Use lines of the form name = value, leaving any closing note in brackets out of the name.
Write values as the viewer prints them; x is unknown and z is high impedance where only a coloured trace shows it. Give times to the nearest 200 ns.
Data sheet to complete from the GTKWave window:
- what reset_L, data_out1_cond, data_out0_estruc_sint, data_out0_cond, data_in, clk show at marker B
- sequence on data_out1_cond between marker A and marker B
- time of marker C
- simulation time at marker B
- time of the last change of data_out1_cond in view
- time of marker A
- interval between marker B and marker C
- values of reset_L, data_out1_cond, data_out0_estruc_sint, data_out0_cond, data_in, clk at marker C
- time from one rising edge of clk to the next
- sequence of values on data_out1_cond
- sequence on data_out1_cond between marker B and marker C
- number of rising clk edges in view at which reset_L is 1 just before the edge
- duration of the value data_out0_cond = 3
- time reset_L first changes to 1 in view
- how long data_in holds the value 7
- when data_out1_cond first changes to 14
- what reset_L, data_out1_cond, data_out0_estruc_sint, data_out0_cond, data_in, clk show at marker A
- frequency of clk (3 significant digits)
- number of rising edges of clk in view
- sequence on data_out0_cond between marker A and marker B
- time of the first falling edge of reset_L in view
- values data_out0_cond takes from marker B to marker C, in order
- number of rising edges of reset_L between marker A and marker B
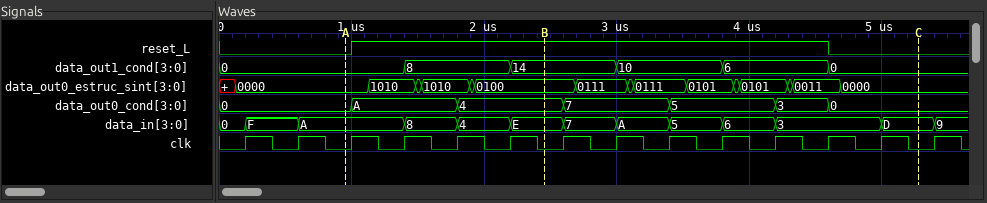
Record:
what reset_L, data_out1_cond, data_out0_estruc_sint, data_out0_cond, data_in, clk show at marker B = reset_L=1, data_out1_cond=14, data_out0_estruc_sint=0100, data_out0_cond=4, data_in=E, clk=0
sequence on data_out1_cond between marker A and marker B = 0, 8, 14
time of marker C = 5200 ns
simulation time at marker B = 2400 ns
time of the last change of data_out1_cond in view = 4600 ns
time of marker A = 1000 ns
interval between marker B and marker C = 2800 ns
values of reset_L, data_out1_cond, data_out0_estruc_sint, data_out0_cond, data_in, clk at marker C = reset_L=0, data_out1_cond=0, data_out0_estruc_sint=0000, data_out0_cond=0, data_in=D, clk=0
time from one rising edge of clk to the next = 400 ns
sequence of values on data_out1_cond = 0, 8, 14, 10, 6, 0
sequence on data_out1_cond between marker B and marker C = 14, 10, 6, 0
number of rising clk edges in view at which reset_L is 1 just before the edge = 9
duration of the value data_out0_cond = 3 = 400 ns
time reset_L first changes to 1 in view = 1000 ns
how long data_in holds the value 7 = 400 ns
when data_out1_cond first changes to 14 = 2200 ns
what reset_L, data_out1_cond, data_out0_estruc_sint, data_out0_cond, data_in, clk show at marker A = reset_L=0, data_out1_cond=0, data_out0_estruc_sint=0000, data_out0_cond=0, data_in=A, clk=0
frequency of clk = 2.50 MHz
number of rising edges of clk in view = 14
sequence on data_out0_cond between marker A and marker B = 0, A, 4
time of the first falling edge of reset_L in view = 4600 ns
values data_out0_cond takes from marker B to marker C, in order = 4, 7, 5, 3, 0
number of rising edges of reset_L between marker A and marker B = 1
